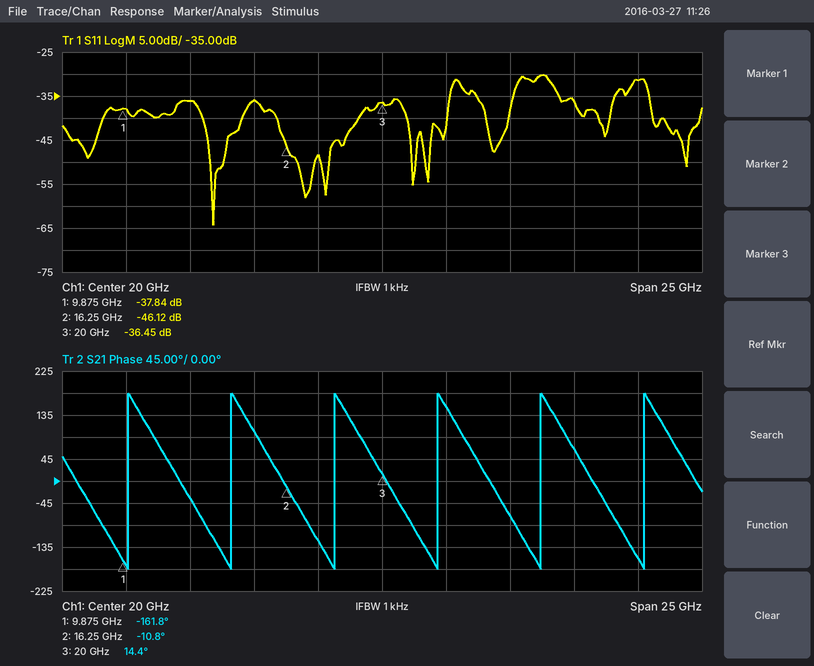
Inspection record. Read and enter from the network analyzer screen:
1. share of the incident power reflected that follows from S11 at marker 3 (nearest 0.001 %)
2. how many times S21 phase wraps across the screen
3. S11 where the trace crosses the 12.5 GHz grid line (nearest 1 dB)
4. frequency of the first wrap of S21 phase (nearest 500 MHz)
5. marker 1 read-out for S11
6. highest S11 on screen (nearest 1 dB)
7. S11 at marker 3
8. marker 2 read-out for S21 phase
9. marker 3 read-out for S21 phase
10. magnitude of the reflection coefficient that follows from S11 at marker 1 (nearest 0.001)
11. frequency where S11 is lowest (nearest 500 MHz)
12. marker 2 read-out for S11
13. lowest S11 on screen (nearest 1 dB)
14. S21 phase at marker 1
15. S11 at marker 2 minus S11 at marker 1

0.023 %
6
-36 dB
10.0 GHz
-37.84 dB
-30 dB
-36.45 dB
-10.8°
14.4°
0.013
13.5 GHz
-46.12 dB
-64 dB
-161.8°
-8.28 dB
